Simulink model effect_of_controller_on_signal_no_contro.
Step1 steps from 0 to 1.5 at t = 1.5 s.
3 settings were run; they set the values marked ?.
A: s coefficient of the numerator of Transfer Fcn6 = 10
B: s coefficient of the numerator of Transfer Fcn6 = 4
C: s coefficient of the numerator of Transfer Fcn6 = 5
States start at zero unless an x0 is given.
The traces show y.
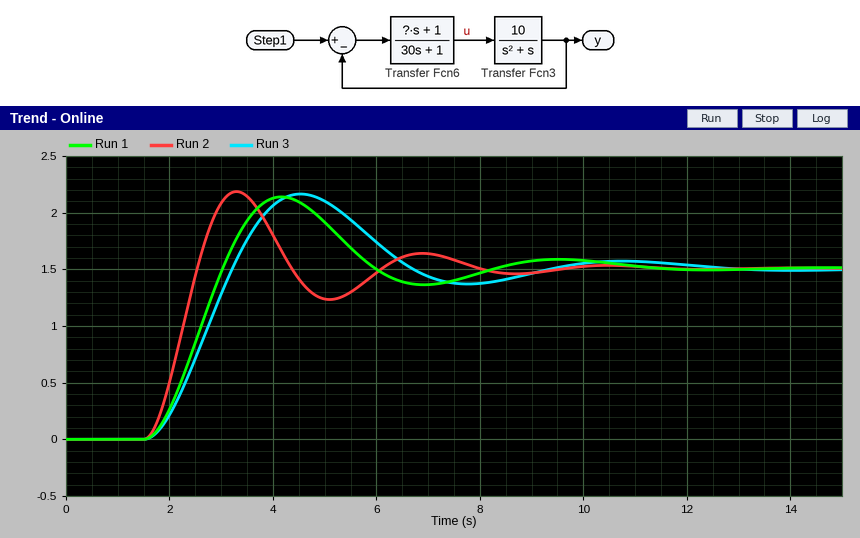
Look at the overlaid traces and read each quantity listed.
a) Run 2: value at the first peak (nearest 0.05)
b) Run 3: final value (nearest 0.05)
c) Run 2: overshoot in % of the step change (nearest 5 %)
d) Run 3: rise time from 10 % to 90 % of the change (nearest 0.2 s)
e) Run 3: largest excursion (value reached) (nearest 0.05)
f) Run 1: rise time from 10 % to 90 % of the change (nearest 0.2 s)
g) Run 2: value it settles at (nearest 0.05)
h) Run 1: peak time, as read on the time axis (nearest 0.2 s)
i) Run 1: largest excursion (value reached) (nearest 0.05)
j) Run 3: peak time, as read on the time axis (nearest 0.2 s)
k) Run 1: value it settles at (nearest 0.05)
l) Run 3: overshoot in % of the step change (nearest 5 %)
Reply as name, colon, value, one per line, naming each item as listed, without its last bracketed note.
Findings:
Run 2: value at the first peak: 2.20
Run 3: final value: 1.50
Run 2: overshoot in % of the step change: 45 %
Run 3: rise time from 10 % to 90 % of the change: 1.2 s
Run 3: largest excursion (value reached): 2.15
Run 1: rise time from 10 % to 90 % of the change: 1.0 s
Run 2: value it settles at: 1.50
Run 1: peak time, as read on the time axis: 4.2 s
Run 1: largest excursion (value reached): 2.15
Run 3: peak time, as read on the time axis: 4.6 s
Run 1: value it settles at: 1.50
Run 3: overshoot in % of the step change: 45 %
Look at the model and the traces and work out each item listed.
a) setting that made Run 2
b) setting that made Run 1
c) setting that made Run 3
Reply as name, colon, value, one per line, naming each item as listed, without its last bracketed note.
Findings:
setting that made Run 2: A
setting that made Run 1: C
setting that made Run 3: B
